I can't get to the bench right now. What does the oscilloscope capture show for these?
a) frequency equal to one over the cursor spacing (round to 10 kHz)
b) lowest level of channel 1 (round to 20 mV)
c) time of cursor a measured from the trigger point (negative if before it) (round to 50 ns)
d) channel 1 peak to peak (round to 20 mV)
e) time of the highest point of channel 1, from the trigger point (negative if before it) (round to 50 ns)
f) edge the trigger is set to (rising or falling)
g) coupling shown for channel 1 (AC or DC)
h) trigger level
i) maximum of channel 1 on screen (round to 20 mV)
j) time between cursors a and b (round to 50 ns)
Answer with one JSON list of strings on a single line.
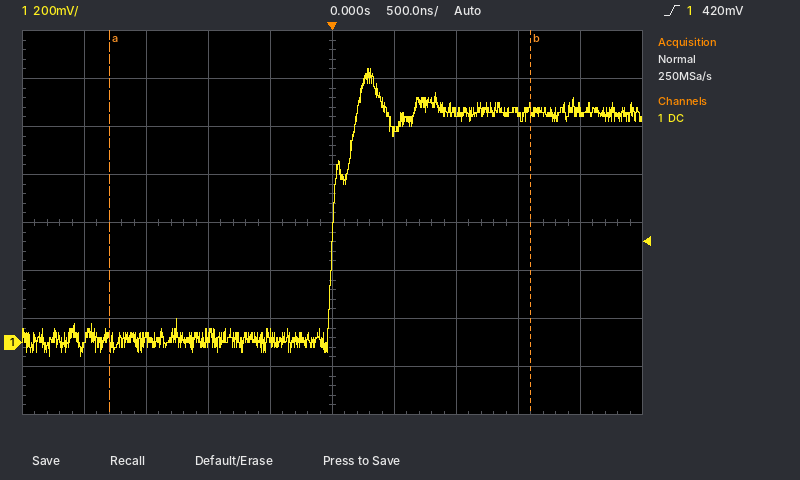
["290 kHz", "-60 mV", "-1.80 µs", "1.20 V", "+300 ns", "rising", "DC", "420 mV", "1.14 V", "3.40 µs"]
